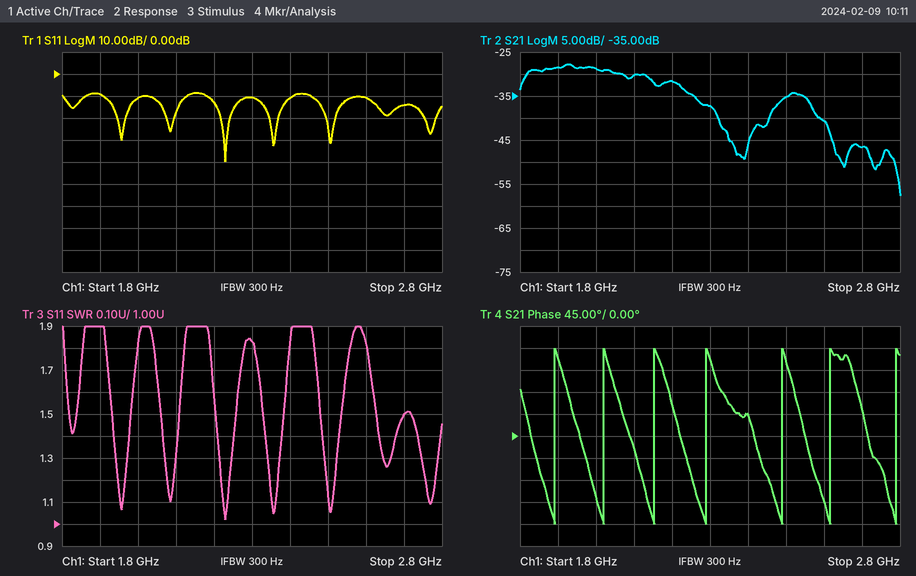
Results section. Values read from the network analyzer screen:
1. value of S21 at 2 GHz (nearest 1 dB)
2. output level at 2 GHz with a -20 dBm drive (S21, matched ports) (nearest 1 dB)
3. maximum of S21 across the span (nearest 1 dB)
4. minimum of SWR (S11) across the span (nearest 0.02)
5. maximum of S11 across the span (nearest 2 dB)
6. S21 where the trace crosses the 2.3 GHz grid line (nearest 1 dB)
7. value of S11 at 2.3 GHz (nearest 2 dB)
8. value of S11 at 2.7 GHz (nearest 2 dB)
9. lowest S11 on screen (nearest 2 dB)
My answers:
-29 dB
-49 dBm
-28 dB
1.02
-8 dB
-37 dB
-10 dB
-14 dB
-40 dB
